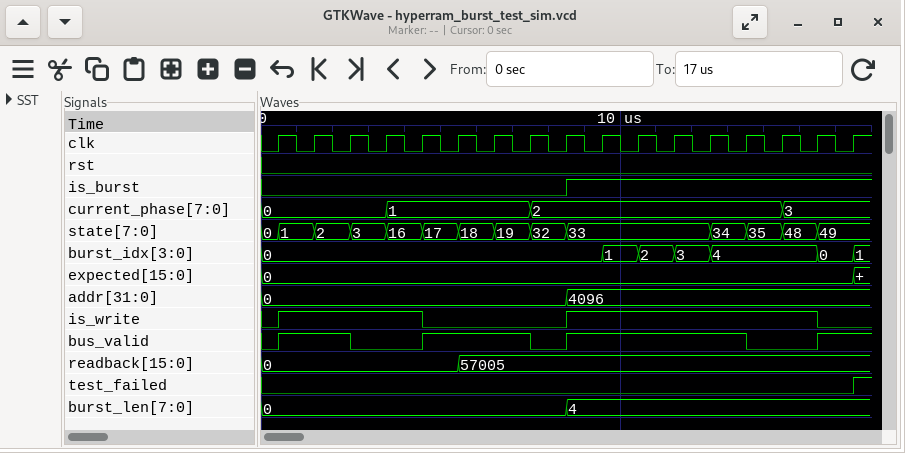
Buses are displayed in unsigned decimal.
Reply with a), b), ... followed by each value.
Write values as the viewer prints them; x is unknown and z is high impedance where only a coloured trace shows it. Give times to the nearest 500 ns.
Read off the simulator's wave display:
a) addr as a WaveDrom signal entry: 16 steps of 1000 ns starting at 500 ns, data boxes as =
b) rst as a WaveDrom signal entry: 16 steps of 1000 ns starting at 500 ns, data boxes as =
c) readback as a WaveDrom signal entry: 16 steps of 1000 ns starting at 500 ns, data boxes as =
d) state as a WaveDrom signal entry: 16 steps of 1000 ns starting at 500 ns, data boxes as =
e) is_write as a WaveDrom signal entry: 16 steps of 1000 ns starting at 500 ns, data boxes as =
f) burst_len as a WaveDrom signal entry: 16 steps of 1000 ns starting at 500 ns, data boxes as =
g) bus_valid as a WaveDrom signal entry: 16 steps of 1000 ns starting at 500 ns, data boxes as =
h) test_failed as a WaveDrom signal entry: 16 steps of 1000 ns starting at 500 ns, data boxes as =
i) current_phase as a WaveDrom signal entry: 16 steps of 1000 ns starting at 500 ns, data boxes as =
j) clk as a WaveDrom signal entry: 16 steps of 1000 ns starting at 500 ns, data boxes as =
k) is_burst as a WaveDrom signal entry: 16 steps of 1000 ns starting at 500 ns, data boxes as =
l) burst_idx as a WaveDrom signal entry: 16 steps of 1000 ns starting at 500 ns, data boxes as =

a) {name: 'addr', wave: '=.......=.......', data: '0 4096'}
b) {name: 'rst', wave: '0...............'}
c) {name: 'readback', wave: '=....=..........', data: '0 57005'}
d) {name: 'state', wave: '=========...====', data: '1 2 3 16 17 18 19 32 33 34 35 48 49'}
e) {name: 'is_write', wave: '1...0...1......0'}
f) {name: 'burst_len', wave: '=.......=.......', data: '0 4'}
g) {name: 'bus_valid', wave: '1.0.1..01....0.1'}
h) {name: 'test_failed', wave: '0...............'}
i) {name: 'current_phase', wave: '=..=...=......=.', data: '0 1 2 3'}
j) {name: 'clk', wave: 'p...............'}
k) {name: 'is_burst', wave: '0.......1.......'}
l) {name: 'burst_idx', wave: '=........====..=', data: '0 1 2 3 4 0'}
